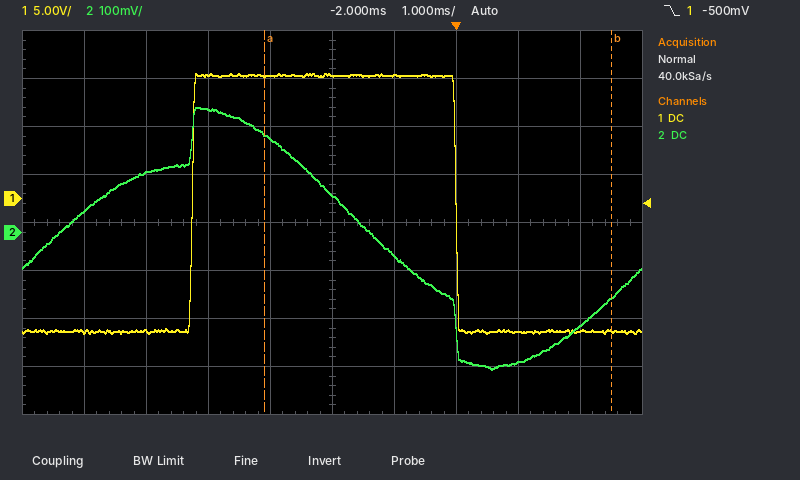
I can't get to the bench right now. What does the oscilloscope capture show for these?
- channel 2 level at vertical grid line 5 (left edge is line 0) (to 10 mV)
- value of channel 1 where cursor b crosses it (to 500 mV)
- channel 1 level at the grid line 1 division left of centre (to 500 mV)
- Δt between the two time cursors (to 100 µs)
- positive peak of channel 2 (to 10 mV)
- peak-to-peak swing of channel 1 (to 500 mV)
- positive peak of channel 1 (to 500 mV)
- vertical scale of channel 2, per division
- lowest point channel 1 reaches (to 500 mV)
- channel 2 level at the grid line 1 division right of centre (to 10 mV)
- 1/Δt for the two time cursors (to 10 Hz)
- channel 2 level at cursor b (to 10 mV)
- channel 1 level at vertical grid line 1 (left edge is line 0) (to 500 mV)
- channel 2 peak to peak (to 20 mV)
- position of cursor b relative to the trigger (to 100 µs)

80 mV
-14.0 V
13.0 V
5.6 ms
260 mV
27.0 V
13.0 V
100 mV
-14.0 V
-50 mV
180 Hz
-140 mV
-14.0 V
540 mV
+2.5 ms
